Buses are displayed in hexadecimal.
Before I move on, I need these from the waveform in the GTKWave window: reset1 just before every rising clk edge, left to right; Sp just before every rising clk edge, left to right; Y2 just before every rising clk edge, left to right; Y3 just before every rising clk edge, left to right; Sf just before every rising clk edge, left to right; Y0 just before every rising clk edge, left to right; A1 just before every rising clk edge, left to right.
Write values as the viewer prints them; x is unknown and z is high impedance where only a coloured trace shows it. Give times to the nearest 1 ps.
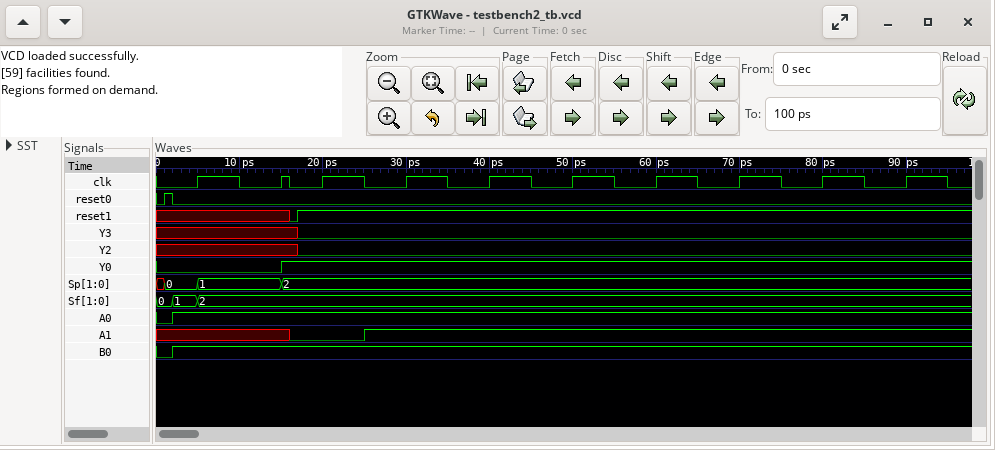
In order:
x x 1 1 1 1 1 1 1 1
0, 1, 2, 2, 2, 2, 2, 2, 2, 2
x x 0 0 0 0 0 0 0 0
x x 0 0 0 0 0 0 0 0
1, 2, 2, 2, 2, 2, 2, 2, 2, 2
0 0 1 1 1 1 1 1 1 1
x x 0 1 1 1 1 1 1 1
